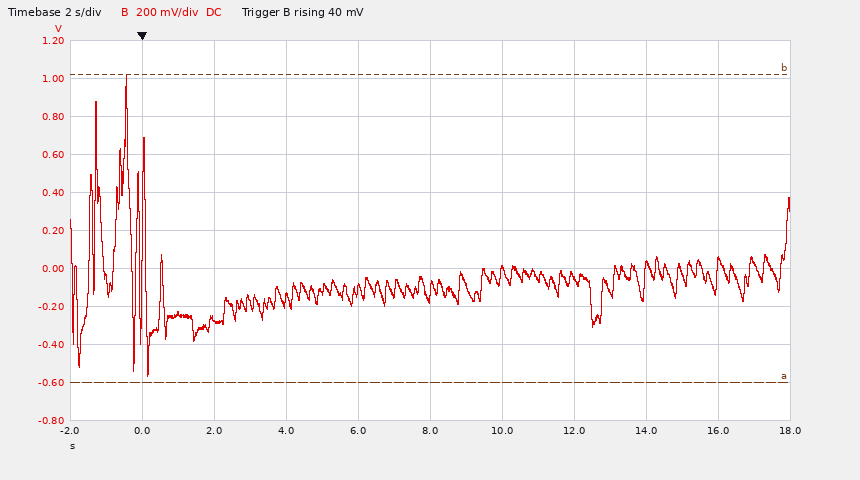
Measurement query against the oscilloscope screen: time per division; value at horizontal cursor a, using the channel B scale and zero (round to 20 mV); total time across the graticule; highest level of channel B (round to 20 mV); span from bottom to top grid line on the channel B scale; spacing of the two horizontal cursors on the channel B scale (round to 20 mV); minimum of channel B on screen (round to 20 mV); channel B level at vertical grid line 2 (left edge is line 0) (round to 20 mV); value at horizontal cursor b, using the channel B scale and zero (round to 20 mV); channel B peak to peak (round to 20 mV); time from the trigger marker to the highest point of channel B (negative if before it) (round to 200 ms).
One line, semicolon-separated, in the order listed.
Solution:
2 s; -600 mV; 20 s; 1.02 V; 2 V; 1.62 V; -560 mV; -260 mV; 1.02 V; 1.58 V; -400 ms
